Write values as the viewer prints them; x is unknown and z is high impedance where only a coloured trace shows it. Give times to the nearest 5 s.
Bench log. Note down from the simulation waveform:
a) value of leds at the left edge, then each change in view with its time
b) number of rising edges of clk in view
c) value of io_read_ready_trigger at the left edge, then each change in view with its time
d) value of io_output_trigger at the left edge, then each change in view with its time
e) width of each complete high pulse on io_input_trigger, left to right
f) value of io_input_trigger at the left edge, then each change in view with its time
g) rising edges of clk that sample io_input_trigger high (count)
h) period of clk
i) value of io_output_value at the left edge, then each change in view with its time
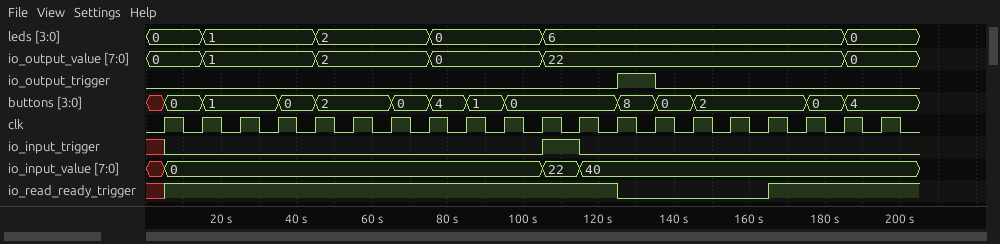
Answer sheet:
0, 1 at 15 s, 2 at 45 s, 0 at 75 s, 6 at 105 s, 0 at 185 s
20
x, 1 at 5 s, 0 at 125 s, 1 at 165 s
0, 1 at 125 s, 0 at 135 s
10 s
x, 0 at 5 s, 1 at 105 s, 0 at 115 s
1
10 s
0, 1 at 15 s, 2 at 45 s, 0 at 75 s, 22 at 105 s, 0 at 185 s
